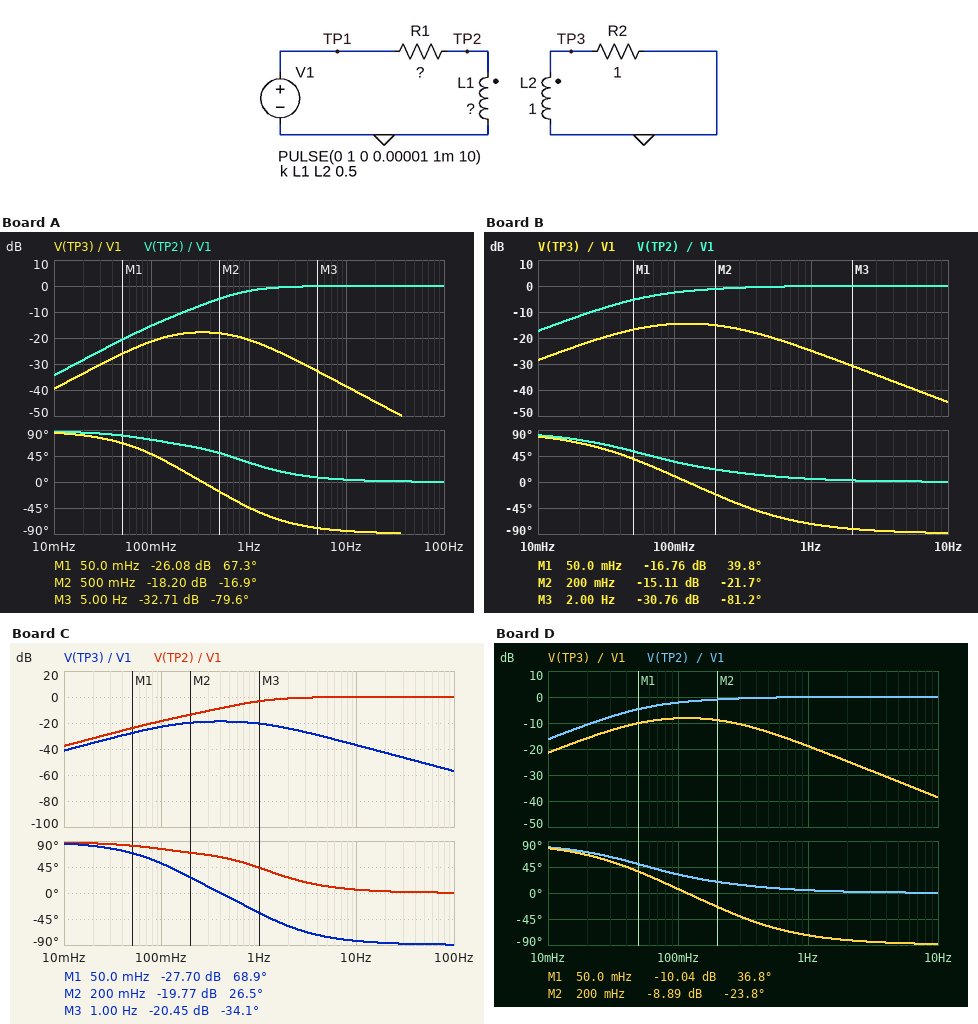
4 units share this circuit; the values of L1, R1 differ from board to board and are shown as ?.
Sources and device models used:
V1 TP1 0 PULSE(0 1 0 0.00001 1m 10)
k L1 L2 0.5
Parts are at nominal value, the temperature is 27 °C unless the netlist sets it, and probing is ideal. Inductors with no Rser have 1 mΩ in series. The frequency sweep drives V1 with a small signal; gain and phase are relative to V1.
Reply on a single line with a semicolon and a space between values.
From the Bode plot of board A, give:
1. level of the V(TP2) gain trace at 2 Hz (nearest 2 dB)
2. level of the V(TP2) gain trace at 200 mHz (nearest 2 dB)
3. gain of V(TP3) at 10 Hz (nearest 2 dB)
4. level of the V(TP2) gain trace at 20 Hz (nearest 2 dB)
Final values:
0 dB; -10 dB; -38 dB; 0 dB
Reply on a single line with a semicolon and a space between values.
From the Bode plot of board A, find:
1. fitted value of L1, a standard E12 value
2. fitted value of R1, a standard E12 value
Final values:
820 mH; 2.7 Ω
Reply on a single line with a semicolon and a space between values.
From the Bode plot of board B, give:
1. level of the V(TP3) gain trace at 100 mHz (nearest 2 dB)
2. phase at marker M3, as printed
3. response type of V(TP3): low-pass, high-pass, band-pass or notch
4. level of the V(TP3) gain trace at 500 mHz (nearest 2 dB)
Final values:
-14 dB; -81.2 deg; band-pass; -20 dB
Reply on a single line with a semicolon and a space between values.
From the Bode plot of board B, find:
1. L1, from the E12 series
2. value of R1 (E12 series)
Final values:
3.3 H; 1.5 Ω
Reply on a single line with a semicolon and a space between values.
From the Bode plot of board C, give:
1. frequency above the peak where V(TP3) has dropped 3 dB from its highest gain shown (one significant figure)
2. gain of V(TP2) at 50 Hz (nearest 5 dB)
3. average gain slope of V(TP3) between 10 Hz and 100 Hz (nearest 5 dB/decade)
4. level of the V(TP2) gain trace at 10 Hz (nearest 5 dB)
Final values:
1 Hz; 0 dB; -20 dB/decade; 0 dB
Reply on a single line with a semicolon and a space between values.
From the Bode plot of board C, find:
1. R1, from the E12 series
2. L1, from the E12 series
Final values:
2.7 Ω; 560 mH
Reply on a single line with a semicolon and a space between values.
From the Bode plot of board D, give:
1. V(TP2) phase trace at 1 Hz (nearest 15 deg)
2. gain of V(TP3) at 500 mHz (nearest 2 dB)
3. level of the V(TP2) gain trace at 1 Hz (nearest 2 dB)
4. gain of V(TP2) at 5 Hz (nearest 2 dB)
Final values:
0 deg; -14 dB; 0 dB; 0 dB
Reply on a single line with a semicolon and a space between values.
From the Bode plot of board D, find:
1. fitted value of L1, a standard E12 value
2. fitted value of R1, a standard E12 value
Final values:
820 mH; 0.33 Ω
